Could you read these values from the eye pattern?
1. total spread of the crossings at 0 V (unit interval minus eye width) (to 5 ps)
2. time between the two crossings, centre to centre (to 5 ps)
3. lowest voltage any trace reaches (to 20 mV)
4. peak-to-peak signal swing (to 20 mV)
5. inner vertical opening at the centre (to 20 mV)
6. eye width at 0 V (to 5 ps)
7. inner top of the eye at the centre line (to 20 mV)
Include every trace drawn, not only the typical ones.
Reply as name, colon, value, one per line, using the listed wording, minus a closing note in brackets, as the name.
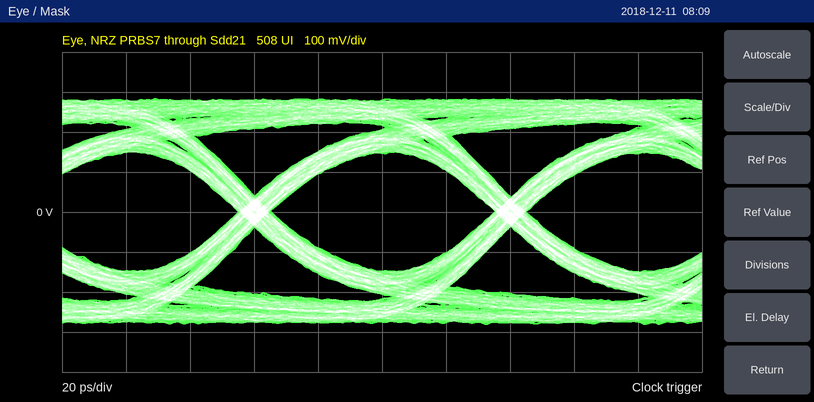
total spread of the crossings at 0 V (unit interval minus eye width): 10 ps
time between the two crossings, centre to centre: 80 ps
lowest voltage any trace reaches: -280 mV
peak-to-peak signal swing: 560 mV
inner vertical opening at the centre: 300 mV
eye width at 0 V: 70 ps
inner top of the eye at the centre line: 140 mV
